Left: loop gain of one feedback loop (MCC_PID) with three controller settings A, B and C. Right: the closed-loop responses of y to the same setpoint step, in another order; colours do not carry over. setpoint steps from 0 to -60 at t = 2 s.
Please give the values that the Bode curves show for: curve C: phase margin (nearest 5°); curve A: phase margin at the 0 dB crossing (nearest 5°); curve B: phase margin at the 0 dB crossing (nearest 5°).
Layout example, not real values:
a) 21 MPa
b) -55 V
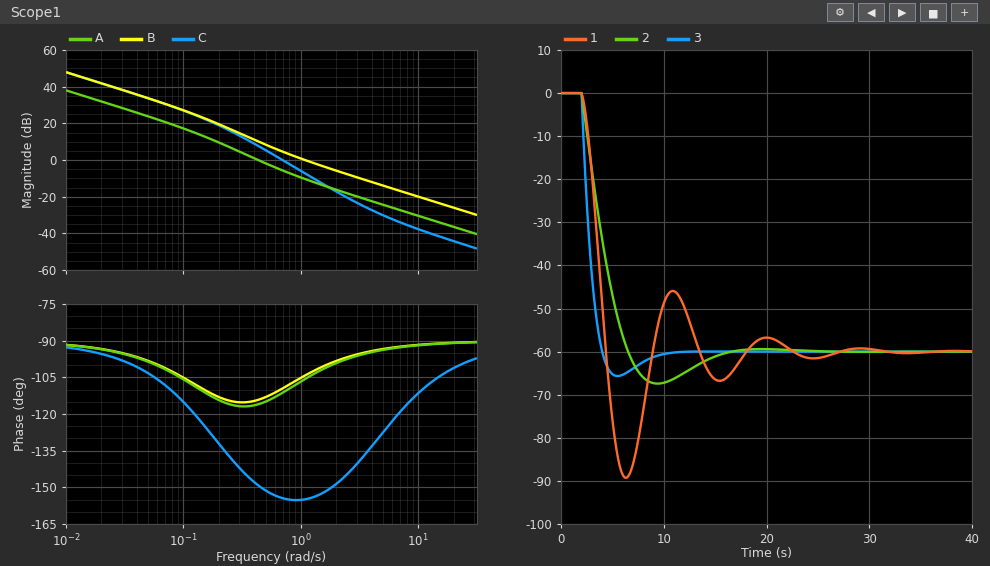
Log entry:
a) 25°
b) 65°
c) 75°
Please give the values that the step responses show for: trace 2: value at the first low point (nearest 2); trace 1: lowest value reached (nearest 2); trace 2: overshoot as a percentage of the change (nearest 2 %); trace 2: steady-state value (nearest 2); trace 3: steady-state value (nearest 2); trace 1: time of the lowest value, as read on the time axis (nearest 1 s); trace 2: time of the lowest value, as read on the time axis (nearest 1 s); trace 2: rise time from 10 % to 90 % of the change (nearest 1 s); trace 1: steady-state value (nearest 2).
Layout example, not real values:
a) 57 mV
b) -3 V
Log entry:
a) -68
b) -90
c) 12 %
d) -60
e) -60
f) 6 s
g) 9 s
h) 3 s
i) -60
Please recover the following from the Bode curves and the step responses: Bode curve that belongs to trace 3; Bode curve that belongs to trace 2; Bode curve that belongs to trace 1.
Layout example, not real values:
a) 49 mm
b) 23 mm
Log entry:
a) B
b) A
c) C
